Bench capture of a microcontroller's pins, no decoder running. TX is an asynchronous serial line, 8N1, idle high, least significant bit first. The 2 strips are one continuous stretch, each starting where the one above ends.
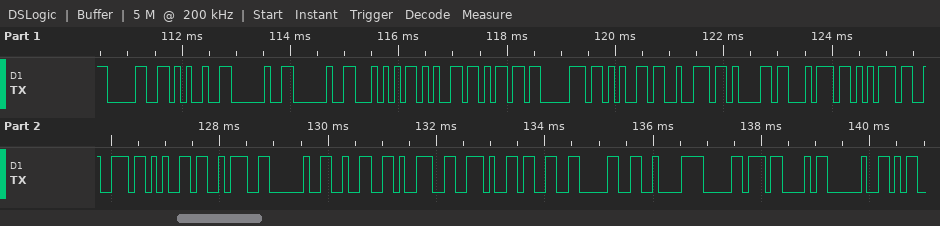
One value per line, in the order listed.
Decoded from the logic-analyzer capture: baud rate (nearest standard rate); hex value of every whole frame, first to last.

9600 baud
30 25 20 20 54 65 6D 70 65 72 61 74 75 72 65 3A 20 32 39 2E 33 30 C2 B0 43 20
